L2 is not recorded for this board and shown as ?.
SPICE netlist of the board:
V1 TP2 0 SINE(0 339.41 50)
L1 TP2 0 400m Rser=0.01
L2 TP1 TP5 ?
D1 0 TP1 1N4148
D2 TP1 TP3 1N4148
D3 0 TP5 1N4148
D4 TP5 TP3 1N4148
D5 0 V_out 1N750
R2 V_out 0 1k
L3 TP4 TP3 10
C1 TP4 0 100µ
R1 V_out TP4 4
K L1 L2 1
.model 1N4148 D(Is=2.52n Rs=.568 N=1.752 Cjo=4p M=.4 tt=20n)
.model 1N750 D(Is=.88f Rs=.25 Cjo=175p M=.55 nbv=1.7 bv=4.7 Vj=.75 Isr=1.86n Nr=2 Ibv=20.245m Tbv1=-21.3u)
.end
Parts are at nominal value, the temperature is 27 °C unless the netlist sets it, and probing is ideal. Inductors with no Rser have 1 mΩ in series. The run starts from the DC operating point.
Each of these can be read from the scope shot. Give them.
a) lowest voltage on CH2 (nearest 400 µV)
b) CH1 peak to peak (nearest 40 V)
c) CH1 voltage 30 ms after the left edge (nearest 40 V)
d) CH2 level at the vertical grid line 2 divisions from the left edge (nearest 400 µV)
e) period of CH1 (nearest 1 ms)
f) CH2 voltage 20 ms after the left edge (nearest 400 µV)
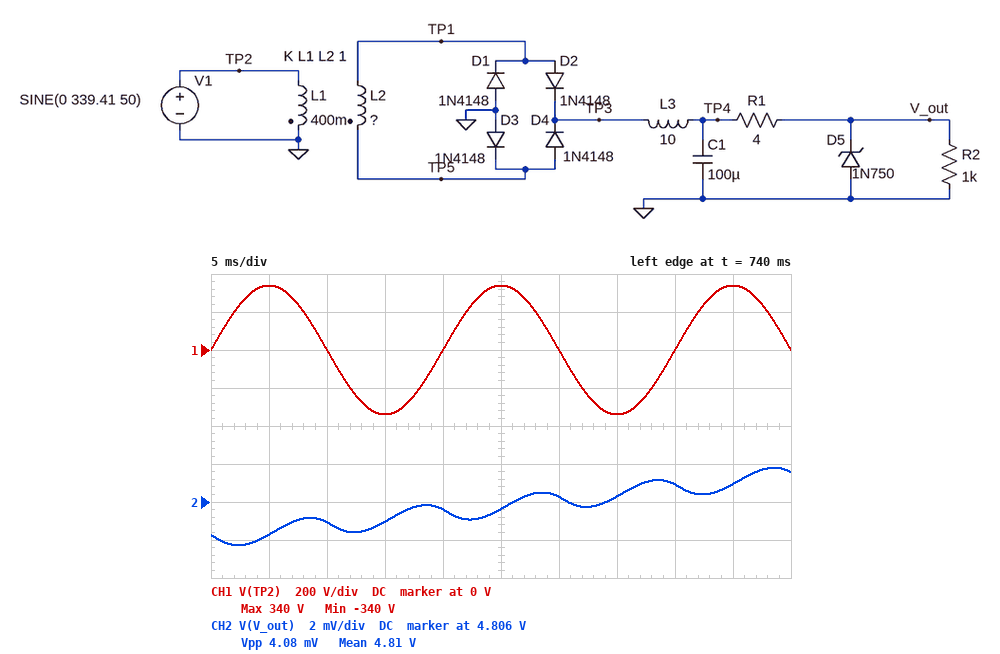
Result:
4.8036 V
680 V
0 V
4.8048 V
20 ms
4.8056 V
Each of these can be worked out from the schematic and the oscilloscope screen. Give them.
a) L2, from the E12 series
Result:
560 µH
